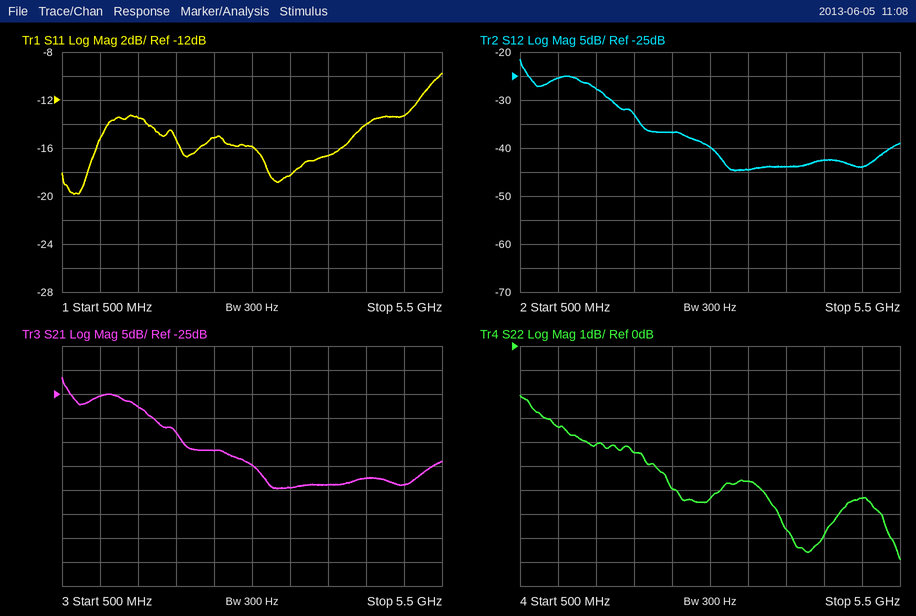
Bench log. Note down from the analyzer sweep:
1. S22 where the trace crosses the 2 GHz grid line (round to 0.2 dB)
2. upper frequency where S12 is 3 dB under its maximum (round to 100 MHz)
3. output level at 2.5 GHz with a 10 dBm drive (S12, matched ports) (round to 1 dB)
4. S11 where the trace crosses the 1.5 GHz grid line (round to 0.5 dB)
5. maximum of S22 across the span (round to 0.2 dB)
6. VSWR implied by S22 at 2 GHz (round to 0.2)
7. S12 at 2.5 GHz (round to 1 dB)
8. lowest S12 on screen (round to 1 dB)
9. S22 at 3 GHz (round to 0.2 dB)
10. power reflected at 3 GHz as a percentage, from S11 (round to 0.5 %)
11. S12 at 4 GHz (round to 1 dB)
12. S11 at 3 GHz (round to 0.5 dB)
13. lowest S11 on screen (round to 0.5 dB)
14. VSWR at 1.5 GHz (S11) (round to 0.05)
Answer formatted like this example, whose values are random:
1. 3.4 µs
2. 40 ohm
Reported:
1. -4.4 dB
2. 600 MHz
3. -27 dBm
4. -13.5 dB
5. -2.0 dB
6. 4.0
7. -37 dB
8. -45 dB
9. -6.4 dB
10. 2.5 %
11. -44 dB
12. -16.0 dB
13. -20.0 dB
14. 1.55
